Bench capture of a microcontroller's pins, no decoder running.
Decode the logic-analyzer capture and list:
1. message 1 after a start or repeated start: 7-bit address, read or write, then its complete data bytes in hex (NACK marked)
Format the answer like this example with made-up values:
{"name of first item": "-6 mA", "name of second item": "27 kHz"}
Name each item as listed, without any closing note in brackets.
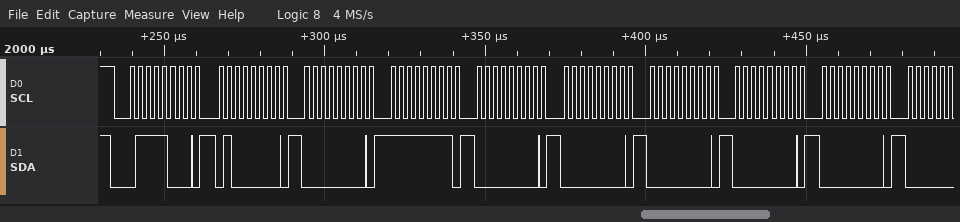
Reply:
{"message 1 after a start or repeated start: 7-bit address, read or write, then its complete data bytes in hex": "0x3C write: 40 00 FF 00 00 00 00 00"}
